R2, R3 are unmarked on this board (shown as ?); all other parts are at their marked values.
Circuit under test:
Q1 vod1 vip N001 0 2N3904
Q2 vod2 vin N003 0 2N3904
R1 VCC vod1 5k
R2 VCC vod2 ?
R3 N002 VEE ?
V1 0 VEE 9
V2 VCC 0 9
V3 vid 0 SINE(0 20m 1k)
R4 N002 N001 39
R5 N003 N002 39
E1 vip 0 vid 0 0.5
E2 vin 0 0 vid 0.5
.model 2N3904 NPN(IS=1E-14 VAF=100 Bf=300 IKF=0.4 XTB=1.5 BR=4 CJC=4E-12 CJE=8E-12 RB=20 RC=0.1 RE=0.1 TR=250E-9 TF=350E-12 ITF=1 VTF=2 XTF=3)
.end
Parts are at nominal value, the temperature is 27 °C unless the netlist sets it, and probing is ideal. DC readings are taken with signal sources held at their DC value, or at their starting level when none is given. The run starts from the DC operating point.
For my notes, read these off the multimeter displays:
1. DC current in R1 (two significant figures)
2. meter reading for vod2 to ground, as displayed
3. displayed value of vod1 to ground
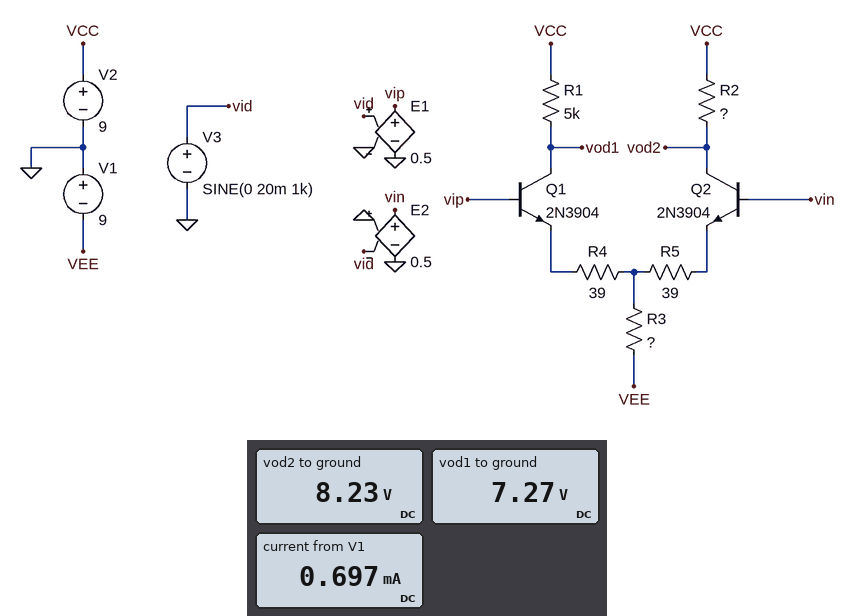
350 µA
8.23 V
7.27 V
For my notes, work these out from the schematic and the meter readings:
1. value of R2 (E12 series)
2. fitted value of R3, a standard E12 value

2.2 kΩ
12 kΩ
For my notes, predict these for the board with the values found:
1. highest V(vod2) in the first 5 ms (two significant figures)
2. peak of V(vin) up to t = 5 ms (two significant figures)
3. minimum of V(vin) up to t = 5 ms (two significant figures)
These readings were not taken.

8.4 V
10 mV
-10 mV
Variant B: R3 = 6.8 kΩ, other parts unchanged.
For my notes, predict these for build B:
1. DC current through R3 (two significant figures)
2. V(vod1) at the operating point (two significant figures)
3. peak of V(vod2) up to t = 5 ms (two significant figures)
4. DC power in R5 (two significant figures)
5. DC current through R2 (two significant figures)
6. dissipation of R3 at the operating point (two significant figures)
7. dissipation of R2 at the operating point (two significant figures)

1.2 mA
6.0 V
7.9 V
15 µW
610 µA
10 mW
830 µW
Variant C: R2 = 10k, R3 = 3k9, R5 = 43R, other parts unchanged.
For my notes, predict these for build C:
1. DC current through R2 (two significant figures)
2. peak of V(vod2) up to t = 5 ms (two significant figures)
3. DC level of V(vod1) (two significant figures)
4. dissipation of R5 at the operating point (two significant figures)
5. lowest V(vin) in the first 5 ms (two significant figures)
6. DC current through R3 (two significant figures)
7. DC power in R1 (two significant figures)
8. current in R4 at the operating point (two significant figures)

960 µA
280 mV
3.4 V
43 µW
-10 mV
2.1 mA
6.4 mW
1.1 mA
